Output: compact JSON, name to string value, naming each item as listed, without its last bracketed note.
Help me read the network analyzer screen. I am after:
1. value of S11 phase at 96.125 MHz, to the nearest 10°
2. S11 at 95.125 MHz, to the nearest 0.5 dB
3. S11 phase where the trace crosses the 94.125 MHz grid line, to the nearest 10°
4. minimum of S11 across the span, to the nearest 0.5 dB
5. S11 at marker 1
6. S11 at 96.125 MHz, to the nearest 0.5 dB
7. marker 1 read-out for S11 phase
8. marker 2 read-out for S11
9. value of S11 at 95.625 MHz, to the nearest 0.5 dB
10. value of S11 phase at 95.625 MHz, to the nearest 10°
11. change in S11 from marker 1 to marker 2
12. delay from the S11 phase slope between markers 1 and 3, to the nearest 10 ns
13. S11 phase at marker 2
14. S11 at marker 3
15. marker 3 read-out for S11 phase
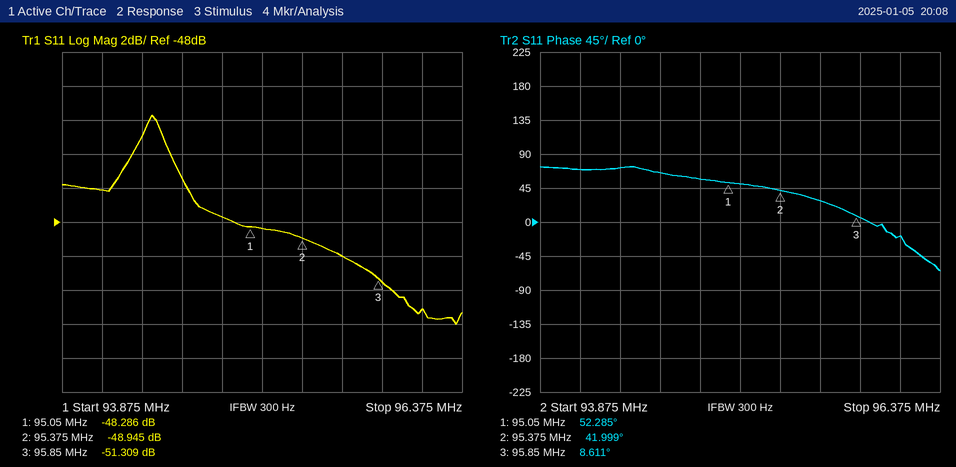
{"value of S11 phase at 96.125 MHz, to the nearest 10°": "-20°", "S11 at 95.125 MHz, to the nearest 0.5 dB": "-48.5 dB", "S11 phase where the trace crosses the 94.125 MHz grid line, to the nearest 10°": "70°", "minimum of S11 across the span, to the nearest 0.5 dB": "-54.0 dB", "S11 at marker 1": "-48.286 dB", "S11 at 96.125 MHz, to the nearest 0.5 dB": "-53.0 dB", "marker 1 read-out for S11 phase": "52.285°", "marker 2 read-out for S11": "-48.945 dB", "value of S11 at 95.625 MHz, to the nearest 0.5 dB": "-50.0 dB", "value of S11 phase at 95.625 MHz, to the nearest 10°": "30°", "change in S11 from marker 1 to marker 2": "-0.659 dB", "delay from the S11 phase slope between markers 1 and 3, to the nearest 10 ns": "150 ns", "S11 phase at marker 2": "41.999°", "S11 at marker 3": "-51.309 dB", "marker 3 read-out for S11 phase": "8.611°"}
